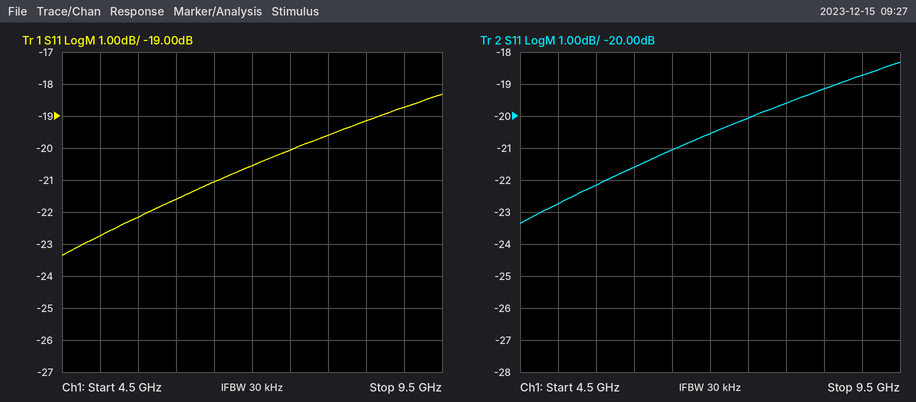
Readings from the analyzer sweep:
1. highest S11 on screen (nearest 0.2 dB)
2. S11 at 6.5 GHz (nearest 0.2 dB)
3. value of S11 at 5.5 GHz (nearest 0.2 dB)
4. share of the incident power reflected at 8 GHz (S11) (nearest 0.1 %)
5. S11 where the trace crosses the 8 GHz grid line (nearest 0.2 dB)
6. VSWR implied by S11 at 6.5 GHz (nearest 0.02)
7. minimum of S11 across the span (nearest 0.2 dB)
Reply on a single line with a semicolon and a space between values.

-18.4 dB; -21.0 dB; -22.2 dB; 1.1 %; -19.6 dB; 1.20; -23.4 dB
